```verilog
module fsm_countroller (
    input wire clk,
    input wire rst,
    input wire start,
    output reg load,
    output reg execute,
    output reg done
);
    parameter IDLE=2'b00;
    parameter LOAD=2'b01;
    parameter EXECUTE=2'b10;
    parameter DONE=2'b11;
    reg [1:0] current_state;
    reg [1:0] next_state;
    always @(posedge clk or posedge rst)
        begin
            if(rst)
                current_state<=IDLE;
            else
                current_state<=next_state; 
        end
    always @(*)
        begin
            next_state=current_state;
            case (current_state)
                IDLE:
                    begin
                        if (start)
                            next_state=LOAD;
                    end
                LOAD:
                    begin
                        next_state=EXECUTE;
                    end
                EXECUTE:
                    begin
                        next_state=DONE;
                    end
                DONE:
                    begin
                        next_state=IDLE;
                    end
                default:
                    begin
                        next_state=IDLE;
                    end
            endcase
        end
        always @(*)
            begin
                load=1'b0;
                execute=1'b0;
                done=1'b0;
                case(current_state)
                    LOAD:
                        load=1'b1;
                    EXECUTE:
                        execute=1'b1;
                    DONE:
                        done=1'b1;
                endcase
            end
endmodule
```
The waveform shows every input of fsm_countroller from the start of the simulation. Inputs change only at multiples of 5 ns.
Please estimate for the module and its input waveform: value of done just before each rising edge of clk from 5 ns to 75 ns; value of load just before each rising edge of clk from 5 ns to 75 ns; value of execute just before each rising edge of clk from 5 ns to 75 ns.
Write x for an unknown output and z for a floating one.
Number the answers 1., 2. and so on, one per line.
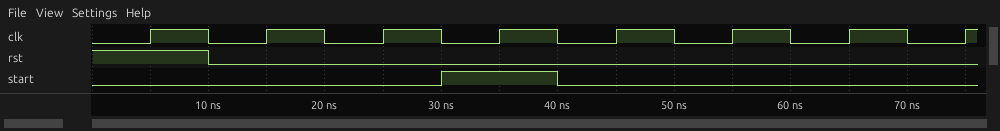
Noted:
1. 0 0 0 0 0 0 1 0
2. 0 0 0 0 1 0 0 0
3. 0 0 0 0 0 1 0 0
